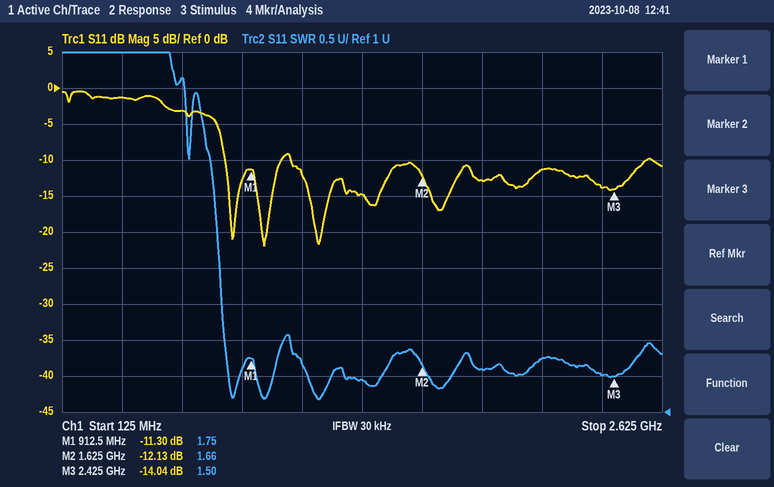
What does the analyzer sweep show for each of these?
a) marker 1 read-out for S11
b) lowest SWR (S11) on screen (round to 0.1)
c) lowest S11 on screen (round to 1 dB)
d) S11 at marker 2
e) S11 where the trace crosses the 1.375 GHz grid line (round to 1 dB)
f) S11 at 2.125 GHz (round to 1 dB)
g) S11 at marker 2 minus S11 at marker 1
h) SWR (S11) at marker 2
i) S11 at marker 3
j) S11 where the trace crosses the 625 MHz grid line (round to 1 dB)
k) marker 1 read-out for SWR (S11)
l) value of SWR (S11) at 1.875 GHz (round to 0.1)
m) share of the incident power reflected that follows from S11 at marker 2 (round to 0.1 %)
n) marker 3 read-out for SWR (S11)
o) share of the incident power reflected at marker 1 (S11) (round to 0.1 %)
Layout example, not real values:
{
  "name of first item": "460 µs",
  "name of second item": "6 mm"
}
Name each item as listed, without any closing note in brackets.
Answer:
{
  "marker 1 read-out for S11": "-11.30 dB",
  "lowest SWR (S11) on screen": "1.2",
  "lowest S11 on screen": "-22 dB",
  "S11 at marker 2": "-12.13 dB",
  "S11 where the trace crosses the 1.375 GHz grid line": "-15 dB",
  "S11 at 2.125 GHz": "-11 dB",
  "S11 at marker 2 minus S11 at marker 1": "-0.83 dB",
  "SWR (S11) at marker 2": "1.66",
  "S11 at marker 3": "-14.04 dB",
  "S11 where the trace crosses the 625 MHz grid line": "-3 dB",
  "marker 1 read-out for SWR": "1.75",
  "value of SWR (S11) at 1.875 GHz": "1.6",
  "share of the incident power reflected that follows from S11 at marker 2": "6.1 %",
  "marker 3 read-out for SWR": "1.50",
  "share of the incident power reflected at marker 1 (S11)": "7.4 %"
}
